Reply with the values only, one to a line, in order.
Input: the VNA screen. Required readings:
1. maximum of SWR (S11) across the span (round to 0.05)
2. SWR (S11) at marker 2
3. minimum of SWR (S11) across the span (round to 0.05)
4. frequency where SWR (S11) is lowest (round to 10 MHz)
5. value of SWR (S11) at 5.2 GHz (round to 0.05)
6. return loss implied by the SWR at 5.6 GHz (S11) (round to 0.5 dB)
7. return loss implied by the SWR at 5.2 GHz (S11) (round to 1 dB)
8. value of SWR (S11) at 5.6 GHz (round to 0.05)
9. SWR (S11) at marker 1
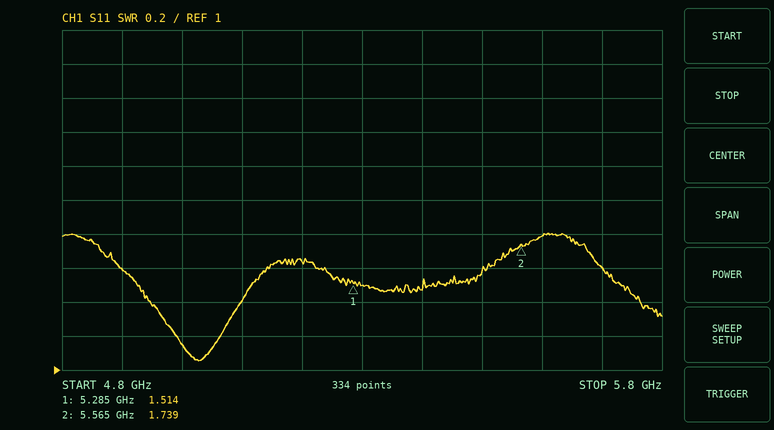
1.80
1.739
1.05
5.03 GHz
1.65
11.0 dB
12 dB
1.80
1.514
